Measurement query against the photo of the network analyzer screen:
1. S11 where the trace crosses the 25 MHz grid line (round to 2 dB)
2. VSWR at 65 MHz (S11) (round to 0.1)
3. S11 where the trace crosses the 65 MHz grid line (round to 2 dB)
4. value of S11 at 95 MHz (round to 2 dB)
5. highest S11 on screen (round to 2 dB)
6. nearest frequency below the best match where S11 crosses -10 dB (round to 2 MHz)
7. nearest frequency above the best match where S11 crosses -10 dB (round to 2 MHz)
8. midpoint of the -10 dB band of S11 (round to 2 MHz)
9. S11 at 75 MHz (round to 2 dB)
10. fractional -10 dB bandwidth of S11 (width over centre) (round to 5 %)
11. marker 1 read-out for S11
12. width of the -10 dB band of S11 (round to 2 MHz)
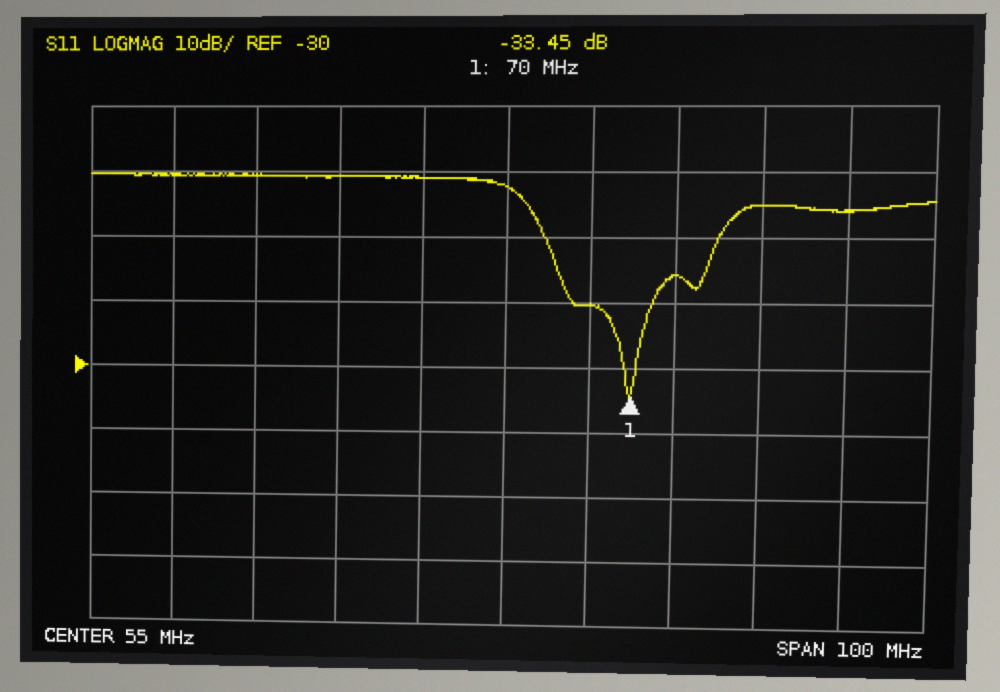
0 dB
1.2
-20 dB
-6 dB
0 dB
60 MHz
80 MHz
70 MHz
-16 dB
30 %
-33.45 dB
20 MHz
